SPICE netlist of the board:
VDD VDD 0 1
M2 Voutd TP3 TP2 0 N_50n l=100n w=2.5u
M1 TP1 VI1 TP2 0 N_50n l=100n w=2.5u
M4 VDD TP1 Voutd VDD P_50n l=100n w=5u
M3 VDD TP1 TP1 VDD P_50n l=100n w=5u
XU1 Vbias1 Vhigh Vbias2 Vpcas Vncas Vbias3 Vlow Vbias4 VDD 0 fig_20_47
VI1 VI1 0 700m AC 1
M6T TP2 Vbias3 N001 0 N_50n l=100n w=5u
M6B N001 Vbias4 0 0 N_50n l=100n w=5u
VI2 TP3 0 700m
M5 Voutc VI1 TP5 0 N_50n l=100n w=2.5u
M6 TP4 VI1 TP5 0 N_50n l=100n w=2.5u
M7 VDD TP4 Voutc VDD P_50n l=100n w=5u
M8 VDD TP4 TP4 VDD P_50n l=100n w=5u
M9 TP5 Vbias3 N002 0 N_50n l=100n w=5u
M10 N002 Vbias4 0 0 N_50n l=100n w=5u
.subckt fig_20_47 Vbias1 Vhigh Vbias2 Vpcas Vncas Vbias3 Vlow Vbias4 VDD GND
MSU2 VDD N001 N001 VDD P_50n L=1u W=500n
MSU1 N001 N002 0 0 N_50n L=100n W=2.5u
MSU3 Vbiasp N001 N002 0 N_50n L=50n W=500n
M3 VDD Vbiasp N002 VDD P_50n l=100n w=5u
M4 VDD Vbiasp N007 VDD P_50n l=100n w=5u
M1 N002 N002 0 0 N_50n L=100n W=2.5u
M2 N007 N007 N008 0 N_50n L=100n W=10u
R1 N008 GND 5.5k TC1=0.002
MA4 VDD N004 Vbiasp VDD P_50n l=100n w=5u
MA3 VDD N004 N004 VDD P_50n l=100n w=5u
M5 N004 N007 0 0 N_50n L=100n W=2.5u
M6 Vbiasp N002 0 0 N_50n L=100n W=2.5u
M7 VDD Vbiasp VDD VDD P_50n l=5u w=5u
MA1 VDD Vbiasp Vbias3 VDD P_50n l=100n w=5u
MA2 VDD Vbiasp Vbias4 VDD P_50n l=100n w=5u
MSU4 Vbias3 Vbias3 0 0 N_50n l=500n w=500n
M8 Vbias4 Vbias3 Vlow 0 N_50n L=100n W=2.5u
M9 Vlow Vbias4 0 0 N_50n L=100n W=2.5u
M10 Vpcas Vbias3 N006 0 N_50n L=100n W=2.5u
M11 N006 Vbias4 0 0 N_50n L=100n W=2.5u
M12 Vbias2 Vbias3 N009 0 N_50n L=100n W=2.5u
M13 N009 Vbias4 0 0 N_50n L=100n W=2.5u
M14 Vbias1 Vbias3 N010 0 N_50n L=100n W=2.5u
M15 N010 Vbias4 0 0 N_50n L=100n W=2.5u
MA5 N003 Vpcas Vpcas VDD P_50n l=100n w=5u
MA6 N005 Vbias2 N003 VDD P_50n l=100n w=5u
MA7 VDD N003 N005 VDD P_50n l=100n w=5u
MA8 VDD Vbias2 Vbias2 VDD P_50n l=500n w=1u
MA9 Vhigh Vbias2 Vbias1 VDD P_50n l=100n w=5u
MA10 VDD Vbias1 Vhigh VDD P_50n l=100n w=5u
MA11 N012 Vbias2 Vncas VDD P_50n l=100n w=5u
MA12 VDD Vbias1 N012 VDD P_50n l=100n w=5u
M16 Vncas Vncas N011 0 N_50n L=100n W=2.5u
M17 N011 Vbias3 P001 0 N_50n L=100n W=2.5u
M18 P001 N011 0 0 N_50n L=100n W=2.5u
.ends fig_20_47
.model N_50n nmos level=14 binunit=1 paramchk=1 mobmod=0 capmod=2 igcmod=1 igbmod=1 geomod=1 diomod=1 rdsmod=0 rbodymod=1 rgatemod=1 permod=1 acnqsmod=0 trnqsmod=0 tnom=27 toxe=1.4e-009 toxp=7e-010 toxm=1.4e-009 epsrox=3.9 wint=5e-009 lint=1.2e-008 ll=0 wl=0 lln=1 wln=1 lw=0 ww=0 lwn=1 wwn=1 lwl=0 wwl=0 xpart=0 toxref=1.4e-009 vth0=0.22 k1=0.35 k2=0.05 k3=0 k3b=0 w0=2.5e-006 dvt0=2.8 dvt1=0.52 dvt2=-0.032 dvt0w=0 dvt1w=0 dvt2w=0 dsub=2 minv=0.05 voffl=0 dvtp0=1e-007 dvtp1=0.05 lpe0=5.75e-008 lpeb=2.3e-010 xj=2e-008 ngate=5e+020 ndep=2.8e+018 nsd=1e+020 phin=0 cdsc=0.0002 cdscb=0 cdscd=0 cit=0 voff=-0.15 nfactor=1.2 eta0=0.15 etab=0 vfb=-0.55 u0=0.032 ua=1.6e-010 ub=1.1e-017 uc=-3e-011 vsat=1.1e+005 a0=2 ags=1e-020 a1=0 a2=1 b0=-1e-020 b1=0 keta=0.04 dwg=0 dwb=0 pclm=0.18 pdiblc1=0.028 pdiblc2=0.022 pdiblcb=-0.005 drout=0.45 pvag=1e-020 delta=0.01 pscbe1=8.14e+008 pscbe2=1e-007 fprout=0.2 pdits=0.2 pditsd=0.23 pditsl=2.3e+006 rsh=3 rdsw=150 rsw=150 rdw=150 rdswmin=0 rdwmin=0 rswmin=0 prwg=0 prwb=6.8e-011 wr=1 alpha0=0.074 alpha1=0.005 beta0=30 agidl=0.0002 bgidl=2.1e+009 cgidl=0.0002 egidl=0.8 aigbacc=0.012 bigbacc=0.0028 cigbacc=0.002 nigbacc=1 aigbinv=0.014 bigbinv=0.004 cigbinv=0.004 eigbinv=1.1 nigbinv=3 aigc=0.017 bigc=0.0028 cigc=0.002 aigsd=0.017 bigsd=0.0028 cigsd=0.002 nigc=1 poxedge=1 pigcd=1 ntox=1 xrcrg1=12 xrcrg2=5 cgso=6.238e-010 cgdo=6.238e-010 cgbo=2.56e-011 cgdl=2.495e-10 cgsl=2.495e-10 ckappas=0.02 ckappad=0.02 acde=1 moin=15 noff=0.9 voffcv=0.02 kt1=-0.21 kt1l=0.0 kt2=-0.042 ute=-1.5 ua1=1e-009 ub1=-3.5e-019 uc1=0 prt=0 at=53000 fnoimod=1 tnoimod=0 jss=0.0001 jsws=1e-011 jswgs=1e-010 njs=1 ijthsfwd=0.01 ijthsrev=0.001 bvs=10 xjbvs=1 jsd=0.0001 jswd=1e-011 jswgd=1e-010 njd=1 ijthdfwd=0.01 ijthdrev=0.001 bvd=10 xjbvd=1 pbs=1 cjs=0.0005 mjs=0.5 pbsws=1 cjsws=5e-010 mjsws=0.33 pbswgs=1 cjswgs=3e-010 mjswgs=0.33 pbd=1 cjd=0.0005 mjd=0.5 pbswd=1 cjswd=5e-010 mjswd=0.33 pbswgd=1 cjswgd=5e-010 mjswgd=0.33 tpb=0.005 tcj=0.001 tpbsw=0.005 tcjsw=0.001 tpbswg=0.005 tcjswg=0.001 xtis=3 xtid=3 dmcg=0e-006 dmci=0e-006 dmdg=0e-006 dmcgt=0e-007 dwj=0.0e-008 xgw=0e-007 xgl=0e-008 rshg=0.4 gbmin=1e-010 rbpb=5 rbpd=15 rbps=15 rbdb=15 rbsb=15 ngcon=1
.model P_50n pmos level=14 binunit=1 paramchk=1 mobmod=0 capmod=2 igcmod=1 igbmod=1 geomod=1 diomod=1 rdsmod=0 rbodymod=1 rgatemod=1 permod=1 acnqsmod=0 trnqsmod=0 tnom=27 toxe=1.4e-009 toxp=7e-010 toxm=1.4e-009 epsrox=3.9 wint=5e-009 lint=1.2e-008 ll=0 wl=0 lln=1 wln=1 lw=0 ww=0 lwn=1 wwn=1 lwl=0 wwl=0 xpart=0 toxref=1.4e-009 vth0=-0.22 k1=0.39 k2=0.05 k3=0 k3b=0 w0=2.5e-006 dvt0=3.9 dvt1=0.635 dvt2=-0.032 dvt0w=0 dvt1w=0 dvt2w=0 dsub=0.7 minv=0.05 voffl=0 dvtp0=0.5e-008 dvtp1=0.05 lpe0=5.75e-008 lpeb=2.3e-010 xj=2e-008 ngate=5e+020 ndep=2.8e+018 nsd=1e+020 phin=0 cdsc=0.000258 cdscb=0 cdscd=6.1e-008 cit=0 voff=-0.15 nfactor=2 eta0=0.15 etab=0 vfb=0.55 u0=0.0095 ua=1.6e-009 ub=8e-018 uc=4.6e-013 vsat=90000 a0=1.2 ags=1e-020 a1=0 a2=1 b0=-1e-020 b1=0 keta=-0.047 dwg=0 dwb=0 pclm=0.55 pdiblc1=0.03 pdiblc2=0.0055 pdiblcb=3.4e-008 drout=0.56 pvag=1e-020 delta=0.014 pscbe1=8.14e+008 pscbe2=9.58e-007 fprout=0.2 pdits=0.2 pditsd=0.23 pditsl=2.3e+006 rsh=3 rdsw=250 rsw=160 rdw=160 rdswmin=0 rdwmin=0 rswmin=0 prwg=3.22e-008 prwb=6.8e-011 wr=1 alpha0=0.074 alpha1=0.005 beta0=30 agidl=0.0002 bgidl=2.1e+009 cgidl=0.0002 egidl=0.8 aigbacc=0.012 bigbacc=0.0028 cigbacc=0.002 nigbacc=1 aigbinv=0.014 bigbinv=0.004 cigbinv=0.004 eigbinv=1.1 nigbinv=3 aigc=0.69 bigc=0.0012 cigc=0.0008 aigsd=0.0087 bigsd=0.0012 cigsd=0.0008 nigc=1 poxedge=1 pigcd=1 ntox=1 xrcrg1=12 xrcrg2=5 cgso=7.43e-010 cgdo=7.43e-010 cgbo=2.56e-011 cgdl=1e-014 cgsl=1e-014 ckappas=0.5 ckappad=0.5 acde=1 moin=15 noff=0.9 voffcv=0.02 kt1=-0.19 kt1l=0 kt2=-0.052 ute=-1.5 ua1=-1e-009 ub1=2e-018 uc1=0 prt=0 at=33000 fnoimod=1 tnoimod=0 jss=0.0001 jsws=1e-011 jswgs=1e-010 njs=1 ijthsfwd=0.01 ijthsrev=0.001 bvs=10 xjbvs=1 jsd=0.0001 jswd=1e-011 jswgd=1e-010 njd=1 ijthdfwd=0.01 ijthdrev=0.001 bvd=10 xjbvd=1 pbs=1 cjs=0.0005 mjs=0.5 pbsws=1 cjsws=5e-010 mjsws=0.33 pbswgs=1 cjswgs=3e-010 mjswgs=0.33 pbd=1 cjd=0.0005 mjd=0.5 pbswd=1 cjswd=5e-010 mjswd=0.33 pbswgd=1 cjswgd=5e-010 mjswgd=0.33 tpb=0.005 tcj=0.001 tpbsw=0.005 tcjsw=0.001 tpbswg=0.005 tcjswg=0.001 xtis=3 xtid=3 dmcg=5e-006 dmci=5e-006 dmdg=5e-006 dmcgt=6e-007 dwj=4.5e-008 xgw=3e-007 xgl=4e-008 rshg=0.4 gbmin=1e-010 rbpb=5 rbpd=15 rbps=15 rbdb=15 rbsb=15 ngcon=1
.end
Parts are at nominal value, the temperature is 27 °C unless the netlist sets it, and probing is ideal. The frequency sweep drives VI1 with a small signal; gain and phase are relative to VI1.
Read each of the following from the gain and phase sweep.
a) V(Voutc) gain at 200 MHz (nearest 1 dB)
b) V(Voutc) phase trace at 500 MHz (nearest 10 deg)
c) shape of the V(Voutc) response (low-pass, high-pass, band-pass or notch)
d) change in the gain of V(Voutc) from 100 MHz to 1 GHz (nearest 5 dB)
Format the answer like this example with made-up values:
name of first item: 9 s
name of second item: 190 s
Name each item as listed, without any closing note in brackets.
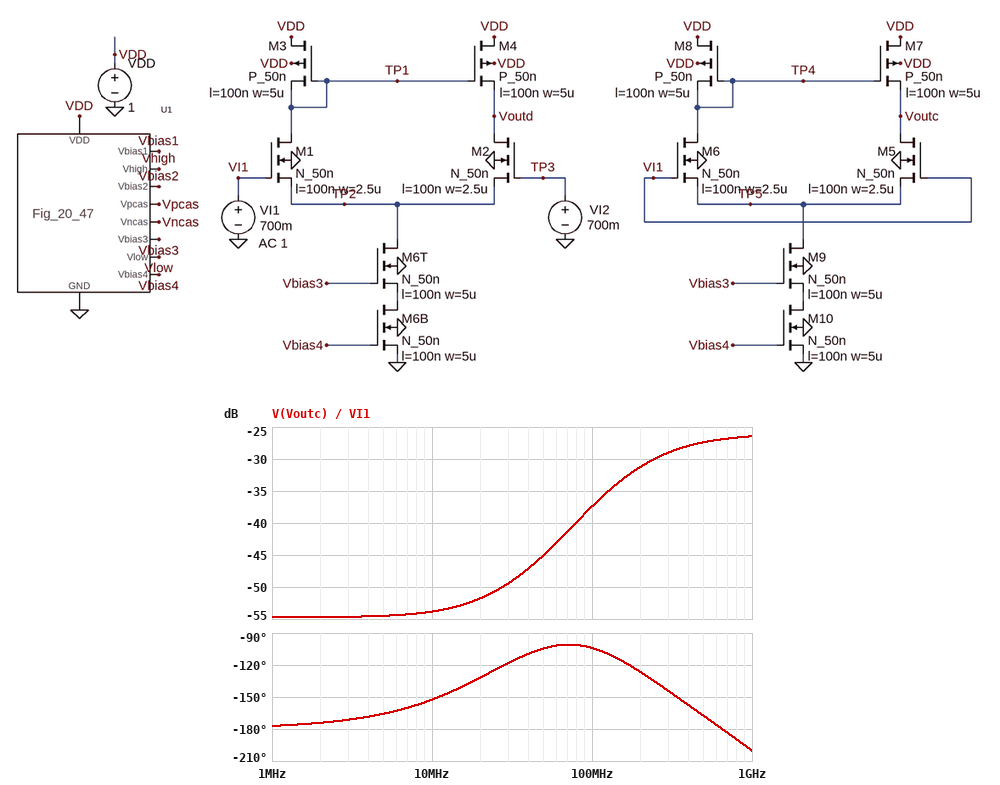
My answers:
V(Voutc) gain at 200 MHz: -31 dB
V(Voutc) phase trace at 500 MHz: -170 deg
shape of the V(Voutc) response: high-pass
change in the gain of V(Voutc) from 100 MHz to 1 GHz: 10 dB
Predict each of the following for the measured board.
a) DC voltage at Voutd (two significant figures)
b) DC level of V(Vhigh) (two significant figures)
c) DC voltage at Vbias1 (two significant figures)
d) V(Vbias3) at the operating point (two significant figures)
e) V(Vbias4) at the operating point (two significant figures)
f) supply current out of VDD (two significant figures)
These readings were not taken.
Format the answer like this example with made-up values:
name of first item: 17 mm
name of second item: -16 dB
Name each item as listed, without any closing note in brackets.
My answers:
DC voltage at Voutd: 650 mV
DC level of V(Vhigh): 790 mV
DC voltage at Vbias1: 640 mV
V(Vbias3) at the operating point: 540 mV
V(Vbias4) at the operating point: 360 mV
supply current out of VDD: 150 µA
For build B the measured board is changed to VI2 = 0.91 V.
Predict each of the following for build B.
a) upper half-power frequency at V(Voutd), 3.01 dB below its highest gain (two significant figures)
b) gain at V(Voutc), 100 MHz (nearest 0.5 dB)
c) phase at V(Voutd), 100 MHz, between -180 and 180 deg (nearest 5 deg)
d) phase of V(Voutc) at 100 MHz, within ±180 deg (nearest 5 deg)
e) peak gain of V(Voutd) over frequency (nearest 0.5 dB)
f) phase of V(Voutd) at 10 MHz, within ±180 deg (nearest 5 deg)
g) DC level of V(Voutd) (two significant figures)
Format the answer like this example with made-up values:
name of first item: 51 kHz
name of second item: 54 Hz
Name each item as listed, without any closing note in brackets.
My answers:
upper half-power frequency at V(Voutd), 3.01 dB below its highest gain: 800 MHz
gain at V(Voutc), 100 MHz: -36.5 dB
phase at V(Voutd), 100 MHz, between -180 and 180 deg: -5 deg
phase of V(Voutc) at 100 MHz, within ±180 deg: -100 deg
peak gain of V(Voutd) over frequency: -1.5 dB
phase of V(Voutd) at 10 MHz, within ±180 deg: 0 deg
DC level of V(Voutd): 290 mV
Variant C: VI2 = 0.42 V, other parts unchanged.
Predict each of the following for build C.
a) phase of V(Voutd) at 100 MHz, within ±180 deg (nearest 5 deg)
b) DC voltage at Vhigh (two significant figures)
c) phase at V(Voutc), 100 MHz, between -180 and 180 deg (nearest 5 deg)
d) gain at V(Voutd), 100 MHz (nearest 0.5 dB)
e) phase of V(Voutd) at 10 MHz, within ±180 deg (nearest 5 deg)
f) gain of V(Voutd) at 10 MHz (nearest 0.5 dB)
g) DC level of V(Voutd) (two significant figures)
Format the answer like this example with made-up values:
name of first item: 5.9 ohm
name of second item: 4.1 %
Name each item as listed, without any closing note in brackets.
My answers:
phase of V(Voutd) at 100 MHz, within ±180 deg: -10 deg
DC voltage at Vhigh: 790 mV
phase at V(Voutc), 100 MHz, between -180 and 180 deg: -100 deg
gain at V(Voutd), 100 MHz: -45.0 dB
phase of V(Voutd) at 10 MHz, within ±180 deg: 0 deg
gain of V(Voutd) at 10 MHz: -45.5 dB
DC level of V(Voutd): 1.0 V
